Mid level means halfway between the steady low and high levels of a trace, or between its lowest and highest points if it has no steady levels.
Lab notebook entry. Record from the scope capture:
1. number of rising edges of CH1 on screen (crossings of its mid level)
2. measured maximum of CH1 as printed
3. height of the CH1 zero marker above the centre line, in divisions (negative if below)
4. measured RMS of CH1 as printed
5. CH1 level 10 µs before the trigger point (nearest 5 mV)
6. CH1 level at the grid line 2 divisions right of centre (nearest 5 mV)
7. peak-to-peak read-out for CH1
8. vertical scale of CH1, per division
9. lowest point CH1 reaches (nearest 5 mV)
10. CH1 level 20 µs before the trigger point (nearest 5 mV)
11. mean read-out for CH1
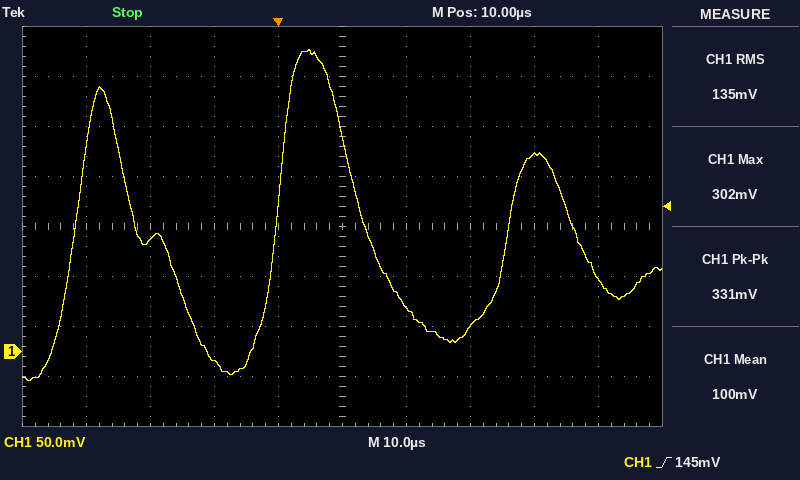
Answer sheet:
3
302 mV
-2.5 div
135 mV
-10 mV
25 mV
331 mV
50 mV
-30 mV
110 mV
100 mV
